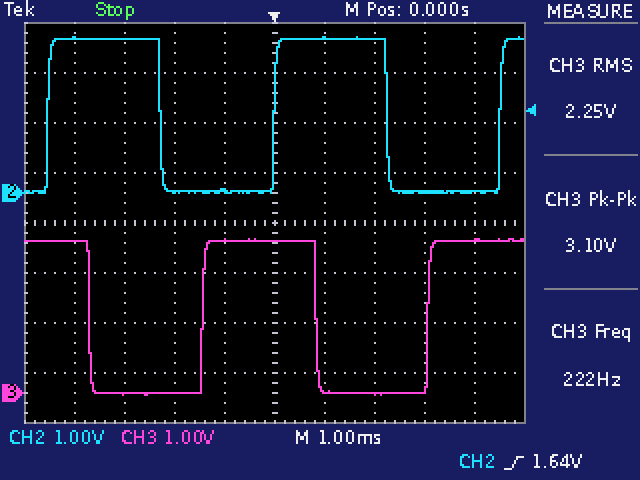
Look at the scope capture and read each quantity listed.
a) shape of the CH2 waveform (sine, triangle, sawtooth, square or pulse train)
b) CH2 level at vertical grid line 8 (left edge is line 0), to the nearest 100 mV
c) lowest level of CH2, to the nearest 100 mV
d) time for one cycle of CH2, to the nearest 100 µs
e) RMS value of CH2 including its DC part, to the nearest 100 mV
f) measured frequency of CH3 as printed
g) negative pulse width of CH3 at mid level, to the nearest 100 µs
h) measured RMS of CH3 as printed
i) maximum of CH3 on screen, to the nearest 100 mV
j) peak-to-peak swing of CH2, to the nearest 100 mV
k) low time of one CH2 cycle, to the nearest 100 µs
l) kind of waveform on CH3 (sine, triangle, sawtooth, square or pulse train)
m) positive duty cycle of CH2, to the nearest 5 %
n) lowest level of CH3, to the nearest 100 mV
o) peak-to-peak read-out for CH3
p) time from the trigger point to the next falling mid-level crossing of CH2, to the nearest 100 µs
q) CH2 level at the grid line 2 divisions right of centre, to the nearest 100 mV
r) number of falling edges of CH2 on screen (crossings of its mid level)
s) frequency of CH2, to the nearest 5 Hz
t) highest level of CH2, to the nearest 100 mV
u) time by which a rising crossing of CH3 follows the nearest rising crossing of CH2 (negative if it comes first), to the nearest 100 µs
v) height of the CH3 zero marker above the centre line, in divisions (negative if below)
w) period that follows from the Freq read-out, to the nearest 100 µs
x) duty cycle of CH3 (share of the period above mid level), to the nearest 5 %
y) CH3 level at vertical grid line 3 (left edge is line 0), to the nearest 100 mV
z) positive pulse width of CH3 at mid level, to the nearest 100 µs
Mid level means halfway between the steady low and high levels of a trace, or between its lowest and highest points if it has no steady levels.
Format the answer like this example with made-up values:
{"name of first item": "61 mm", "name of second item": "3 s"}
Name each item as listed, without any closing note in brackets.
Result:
{"shape of the CH2 waveform": "square", "CH2 level at vertical grid line 8 (left edge is line 0), to the nearest 100 mV": "0.0 V", "lowest level of CH2, to the nearest 100 mV": "0.0 V", "time for one cycle of CH2, to the nearest 100 µs": "4.5 ms", "RMS value of CH2 including its DC part, to the nearest 100 mV": "2.2 V", "measured frequency of CH3 as printed": "222 Hz", "negative pulse width of CH3 at mid level, to the nearest 100 µs": "2.2 ms", "measured RMS of CH3 as printed": "2.25 V", "maximum of CH3 on screen, to the nearest 100 mV": "3.1 V", "peak-to-peak swing of CH2, to the nearest 100 mV": "3.1 V", "low time of one CH2 cycle, to the nearest 100 µs": "2.3 ms", "kind of waveform on CH3": "square", "positive duty cycle of CH2, to the nearest 5 %": "50 %", "lowest level of CH3, to the nearest 100 mV": "0.0 V", "peak-to-peak read-out for CH3": "3.10 V", "time from the trigger point to the next falling mid-level crossing of CH2, to the nearest 100 µs": "2.3 ms", "CH2 level at the grid line 2 divisions right of centre, to the nearest 100 mV": "3.1 V", "number of falling edges of CH2 on screen": "2", "frequency of CH2, to the nearest 5 Hz": "220 Hz", "highest level of CH2, to the nearest 100 mV": "3.1 V", "time by which a rising crossing of CH3 follows the nearest rising crossing of CH2 (negative if it comes first), to the nearest 100 µs": "-1.4 ms", "height of the CH3 zero marker above the centre line, in divisions": "-3.4 div", "period that follows from the Freq read-out, to the nearest 100 µs": "4.5 ms", "duty cycle of CH3 (share of the period above mid level), to the nearest 5 %": "50 %", "CH3 level at vertical grid line 3 (left edge is line 0), to the nearest 100 mV": "0.0 V", "positive pulse width of CH3 at mid level, to the nearest 100 µs": "2.3 ms"}
